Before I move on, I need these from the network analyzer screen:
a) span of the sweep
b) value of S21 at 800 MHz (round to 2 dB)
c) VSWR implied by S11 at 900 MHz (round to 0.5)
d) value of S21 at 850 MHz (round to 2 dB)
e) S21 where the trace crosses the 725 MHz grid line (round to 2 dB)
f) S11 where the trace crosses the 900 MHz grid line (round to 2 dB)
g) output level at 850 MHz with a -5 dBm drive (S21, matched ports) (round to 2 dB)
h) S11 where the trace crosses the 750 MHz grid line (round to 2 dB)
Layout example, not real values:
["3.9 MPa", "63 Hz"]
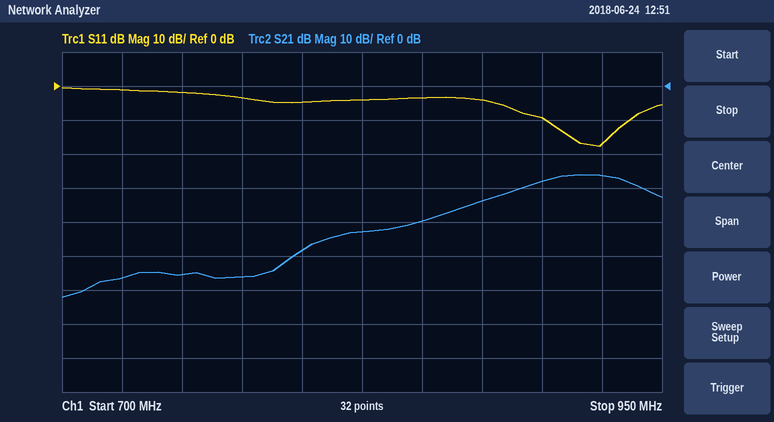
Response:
["250 MHz", "-48 dB", "2.0", "-40 dB", "-56 dB", "-10 dB", "-44 dBm", "-2 dB"]
